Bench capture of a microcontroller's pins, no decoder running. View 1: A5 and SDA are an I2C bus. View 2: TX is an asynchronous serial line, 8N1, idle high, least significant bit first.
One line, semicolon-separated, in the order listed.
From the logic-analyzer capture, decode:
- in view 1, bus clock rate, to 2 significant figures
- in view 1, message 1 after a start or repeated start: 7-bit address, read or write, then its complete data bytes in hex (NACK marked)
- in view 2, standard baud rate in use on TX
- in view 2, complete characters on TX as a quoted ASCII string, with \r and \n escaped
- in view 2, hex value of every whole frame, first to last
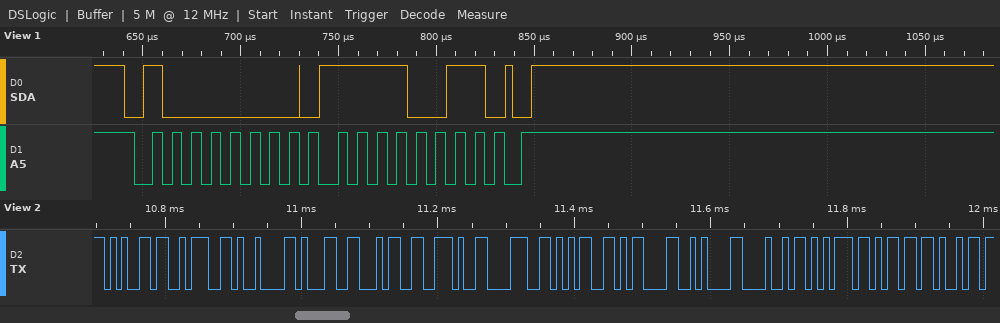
100 kHz; 0x40 write: F3; 115200 baud; "e:\t14.85\r\nHumi"; 0x65 0x3A 0x09 0x31 0x34 0x2E 0x38 0x35 0x0D 0x0A 0x48 0x75 0x6D 0x69
